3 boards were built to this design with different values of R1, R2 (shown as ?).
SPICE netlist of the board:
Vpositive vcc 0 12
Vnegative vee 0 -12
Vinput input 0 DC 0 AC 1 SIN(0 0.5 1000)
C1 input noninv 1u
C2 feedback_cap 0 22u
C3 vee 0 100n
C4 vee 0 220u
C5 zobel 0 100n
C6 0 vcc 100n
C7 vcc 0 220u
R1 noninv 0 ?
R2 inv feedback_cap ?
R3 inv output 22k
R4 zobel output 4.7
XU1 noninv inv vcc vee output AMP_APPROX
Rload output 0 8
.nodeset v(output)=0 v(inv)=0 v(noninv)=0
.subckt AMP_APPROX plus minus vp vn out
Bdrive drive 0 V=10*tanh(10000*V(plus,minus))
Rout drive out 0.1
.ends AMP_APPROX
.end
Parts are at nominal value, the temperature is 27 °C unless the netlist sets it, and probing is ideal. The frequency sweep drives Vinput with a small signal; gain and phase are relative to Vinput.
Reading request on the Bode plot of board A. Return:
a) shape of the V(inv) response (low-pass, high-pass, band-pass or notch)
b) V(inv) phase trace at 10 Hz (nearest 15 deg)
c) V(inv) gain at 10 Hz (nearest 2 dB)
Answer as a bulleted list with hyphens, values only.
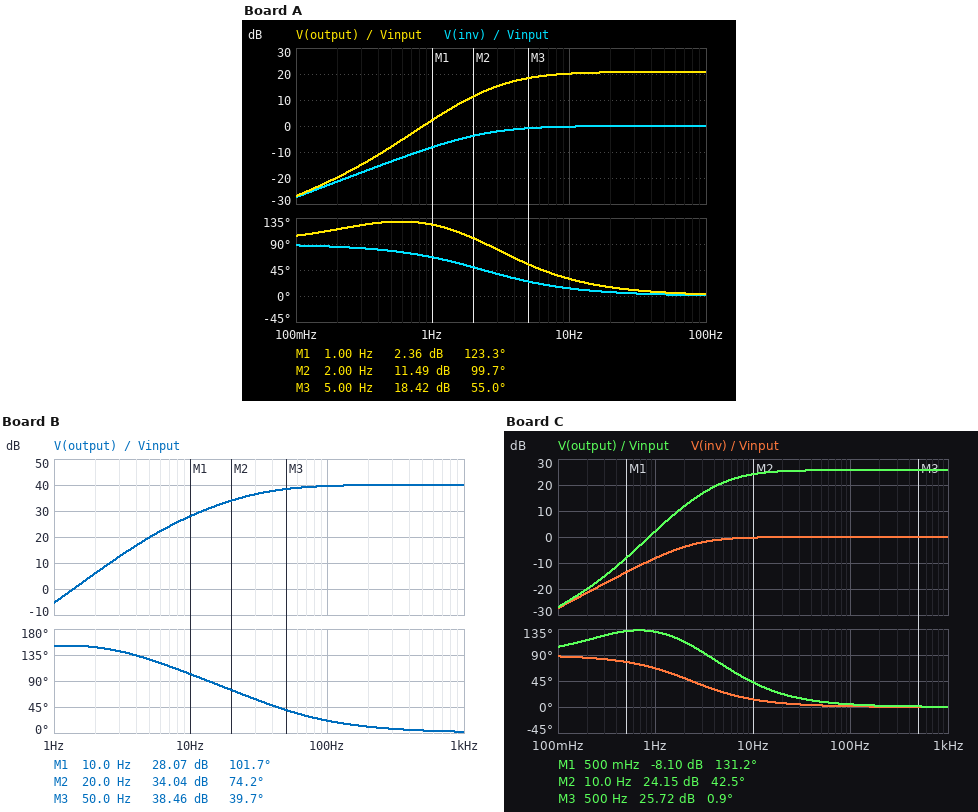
- high-pass
- 15 deg
- 0 dB
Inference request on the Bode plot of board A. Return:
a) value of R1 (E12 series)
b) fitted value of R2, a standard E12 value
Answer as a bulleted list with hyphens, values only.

- 68 kΩ
- 2.2 kΩ
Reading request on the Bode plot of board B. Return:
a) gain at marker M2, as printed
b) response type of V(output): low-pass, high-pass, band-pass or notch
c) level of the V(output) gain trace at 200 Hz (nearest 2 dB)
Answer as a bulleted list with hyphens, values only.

- 34.04 dB
- high-pass
- 40 dB
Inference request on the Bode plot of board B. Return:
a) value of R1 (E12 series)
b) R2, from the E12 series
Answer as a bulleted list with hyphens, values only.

- 27 kΩ
- 220 Ω
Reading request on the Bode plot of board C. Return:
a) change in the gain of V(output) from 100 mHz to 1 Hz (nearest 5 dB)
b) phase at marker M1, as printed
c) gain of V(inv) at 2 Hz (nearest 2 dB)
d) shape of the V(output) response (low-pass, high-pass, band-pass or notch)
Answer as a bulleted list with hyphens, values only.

- 30 dB
- 131.2 deg
- -4 dB
- high-pass
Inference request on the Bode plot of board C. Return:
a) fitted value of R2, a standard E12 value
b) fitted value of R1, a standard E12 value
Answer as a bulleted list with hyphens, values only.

- 1.2 kΩ
- 68 kΩ
